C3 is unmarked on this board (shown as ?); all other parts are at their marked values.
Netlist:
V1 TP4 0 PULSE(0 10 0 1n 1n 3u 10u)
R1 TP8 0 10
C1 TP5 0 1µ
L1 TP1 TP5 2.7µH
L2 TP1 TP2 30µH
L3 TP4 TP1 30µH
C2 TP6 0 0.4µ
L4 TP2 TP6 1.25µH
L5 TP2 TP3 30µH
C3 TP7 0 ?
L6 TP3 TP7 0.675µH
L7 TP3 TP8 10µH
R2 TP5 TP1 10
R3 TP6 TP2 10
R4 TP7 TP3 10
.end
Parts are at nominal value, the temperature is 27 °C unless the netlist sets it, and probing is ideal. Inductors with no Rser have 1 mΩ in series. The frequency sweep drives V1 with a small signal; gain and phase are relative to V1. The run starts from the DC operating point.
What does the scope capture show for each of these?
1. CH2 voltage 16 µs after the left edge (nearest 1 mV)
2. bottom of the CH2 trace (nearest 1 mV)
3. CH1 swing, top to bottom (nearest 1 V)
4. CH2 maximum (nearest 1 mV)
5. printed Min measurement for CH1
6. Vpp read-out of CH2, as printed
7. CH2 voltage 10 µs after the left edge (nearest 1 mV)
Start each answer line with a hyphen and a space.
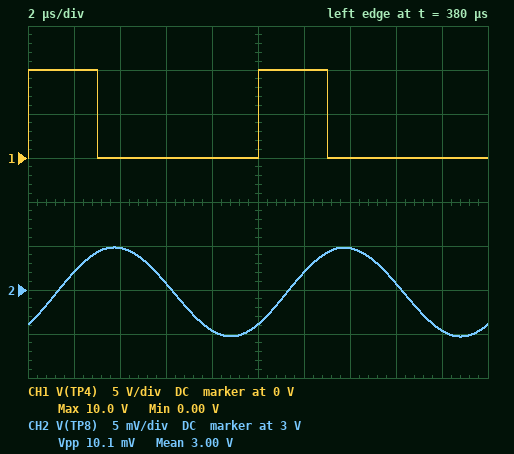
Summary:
- 3.001 V
- 2.995 V
- 10 V
- 3.005 V
- 0.00 V
- 10.1 mV
- 2.996 V
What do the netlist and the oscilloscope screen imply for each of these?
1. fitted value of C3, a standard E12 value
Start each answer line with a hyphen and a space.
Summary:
- 390 nF
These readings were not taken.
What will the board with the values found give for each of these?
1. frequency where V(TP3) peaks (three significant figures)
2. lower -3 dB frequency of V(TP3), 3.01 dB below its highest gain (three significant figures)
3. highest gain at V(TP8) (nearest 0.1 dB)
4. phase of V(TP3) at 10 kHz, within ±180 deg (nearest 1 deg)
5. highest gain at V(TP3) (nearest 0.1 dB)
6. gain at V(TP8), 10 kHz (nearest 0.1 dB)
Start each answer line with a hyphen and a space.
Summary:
- 23.9 kHz
- 9.40 kHz
- 4.1 dB
- -36 deg
- 4.2 dB
- 1.3 dB
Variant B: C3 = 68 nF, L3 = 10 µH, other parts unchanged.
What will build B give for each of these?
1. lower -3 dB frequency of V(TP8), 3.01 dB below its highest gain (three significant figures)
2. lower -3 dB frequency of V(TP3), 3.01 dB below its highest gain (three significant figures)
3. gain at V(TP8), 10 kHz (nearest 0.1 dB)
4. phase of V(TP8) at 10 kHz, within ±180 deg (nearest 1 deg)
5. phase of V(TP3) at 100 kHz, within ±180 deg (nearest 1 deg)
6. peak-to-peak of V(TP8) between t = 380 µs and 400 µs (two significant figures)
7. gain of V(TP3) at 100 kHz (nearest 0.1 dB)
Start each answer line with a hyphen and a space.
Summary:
- 35.9 kHz
- 36.0 kHz
- 0 dB
- -28 deg
- 60 deg
- 54 mV
- -44.2 dB
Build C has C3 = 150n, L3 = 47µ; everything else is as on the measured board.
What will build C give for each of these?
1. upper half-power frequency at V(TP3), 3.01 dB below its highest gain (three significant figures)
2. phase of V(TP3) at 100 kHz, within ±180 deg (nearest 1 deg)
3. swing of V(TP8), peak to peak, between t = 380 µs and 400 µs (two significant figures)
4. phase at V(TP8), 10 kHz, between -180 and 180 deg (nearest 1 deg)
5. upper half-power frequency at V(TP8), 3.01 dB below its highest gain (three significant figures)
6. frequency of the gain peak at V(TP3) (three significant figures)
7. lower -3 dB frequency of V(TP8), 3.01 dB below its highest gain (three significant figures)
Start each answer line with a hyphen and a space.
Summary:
- 27.3 kHz
- 25 deg
- 16 mV
- -44 deg
- 27.2 kHz
- 21.1 kHz
- 9.39 kHz
